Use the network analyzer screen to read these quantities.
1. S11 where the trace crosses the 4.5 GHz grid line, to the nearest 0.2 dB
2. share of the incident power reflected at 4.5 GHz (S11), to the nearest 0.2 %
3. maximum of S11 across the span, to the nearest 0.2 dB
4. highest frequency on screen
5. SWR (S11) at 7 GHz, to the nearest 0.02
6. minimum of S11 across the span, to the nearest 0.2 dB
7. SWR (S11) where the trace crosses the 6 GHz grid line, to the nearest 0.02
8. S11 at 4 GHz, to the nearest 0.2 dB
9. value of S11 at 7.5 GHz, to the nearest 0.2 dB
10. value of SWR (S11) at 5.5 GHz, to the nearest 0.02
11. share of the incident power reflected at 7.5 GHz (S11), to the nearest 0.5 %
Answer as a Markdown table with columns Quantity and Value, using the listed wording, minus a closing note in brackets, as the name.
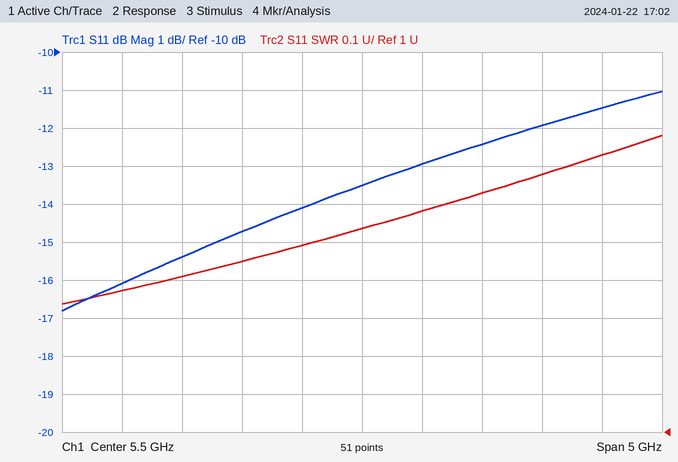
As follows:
| Quantity | Value |
|---|---|
| S11 where the trace crosses the 4.5 GHz grid line, to the nearest 0.2 dB | -14.8 dB |
| share of the incident power reflected at 4.5 GHz (S11), to the nearest 0.2 % | 3.4 % |
| maximum of S11 across the span, to the nearest 0.2 dB | -11.0 dB |
| highest frequency on screen | 8 GHz |
| SWR (S11) at 7 GHz, to the nearest 0.02 | 1.68 |
| minimum of S11 across the span, to the nearest 0.2 dB | -16.8 dB |
| SWR (S11) where the trace crosses the 6 GHz grid line, to the nearest 0.02 | 1.58 |
| S11 at 4 GHz, to the nearest 0.2 dB | -15.4 dB |
| value of S11 at 7.5 GHz, to the nearest 0.2 dB | -11.4 dB |
| value of SWR (S11) at 5.5 GHz, to the nearest 0.02 | 1.54 |
| share of the incident power reflected at 7.5 GHz (S11), to the nearest 0.5 % | 7.0 % |
